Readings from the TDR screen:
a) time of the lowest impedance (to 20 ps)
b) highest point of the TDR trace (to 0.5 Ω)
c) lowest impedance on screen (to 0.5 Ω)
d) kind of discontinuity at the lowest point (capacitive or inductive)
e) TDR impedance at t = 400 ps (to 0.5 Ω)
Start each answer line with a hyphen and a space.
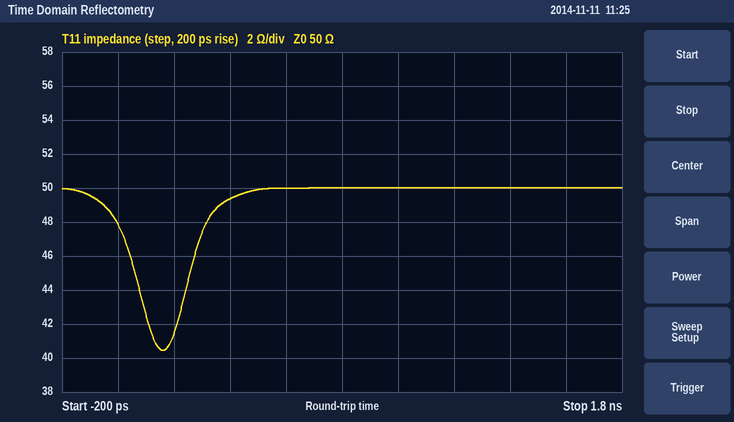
- 160 ps
- 50.0 Ω
- 40.5 Ω
- capacitive
- 49.5 Ω
